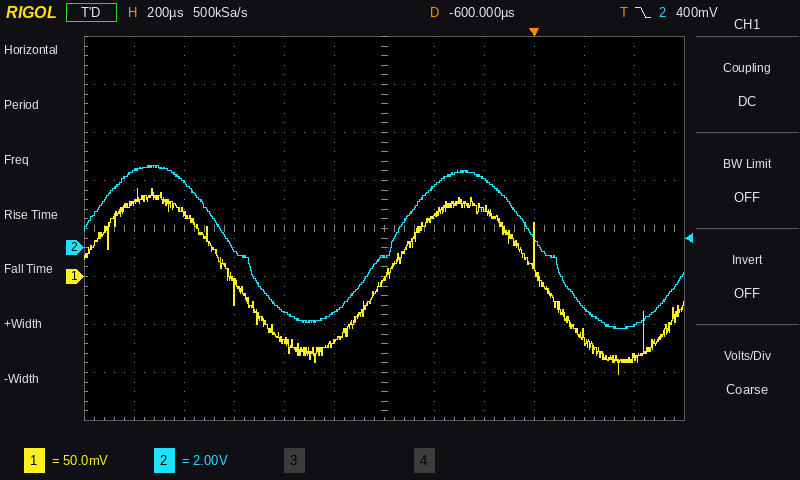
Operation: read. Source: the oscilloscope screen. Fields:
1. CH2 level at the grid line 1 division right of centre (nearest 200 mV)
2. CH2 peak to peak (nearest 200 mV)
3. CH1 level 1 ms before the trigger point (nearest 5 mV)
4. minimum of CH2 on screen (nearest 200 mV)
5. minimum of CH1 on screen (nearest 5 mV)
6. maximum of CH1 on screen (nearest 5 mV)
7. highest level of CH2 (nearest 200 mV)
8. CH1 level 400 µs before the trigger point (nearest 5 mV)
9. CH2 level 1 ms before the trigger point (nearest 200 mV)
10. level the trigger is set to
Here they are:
2.6 V
6.8 V
-65 mV
-3.4 V
-100 mV
90 mV
3.4 V
65 mV
-2.6 V
400 mV
